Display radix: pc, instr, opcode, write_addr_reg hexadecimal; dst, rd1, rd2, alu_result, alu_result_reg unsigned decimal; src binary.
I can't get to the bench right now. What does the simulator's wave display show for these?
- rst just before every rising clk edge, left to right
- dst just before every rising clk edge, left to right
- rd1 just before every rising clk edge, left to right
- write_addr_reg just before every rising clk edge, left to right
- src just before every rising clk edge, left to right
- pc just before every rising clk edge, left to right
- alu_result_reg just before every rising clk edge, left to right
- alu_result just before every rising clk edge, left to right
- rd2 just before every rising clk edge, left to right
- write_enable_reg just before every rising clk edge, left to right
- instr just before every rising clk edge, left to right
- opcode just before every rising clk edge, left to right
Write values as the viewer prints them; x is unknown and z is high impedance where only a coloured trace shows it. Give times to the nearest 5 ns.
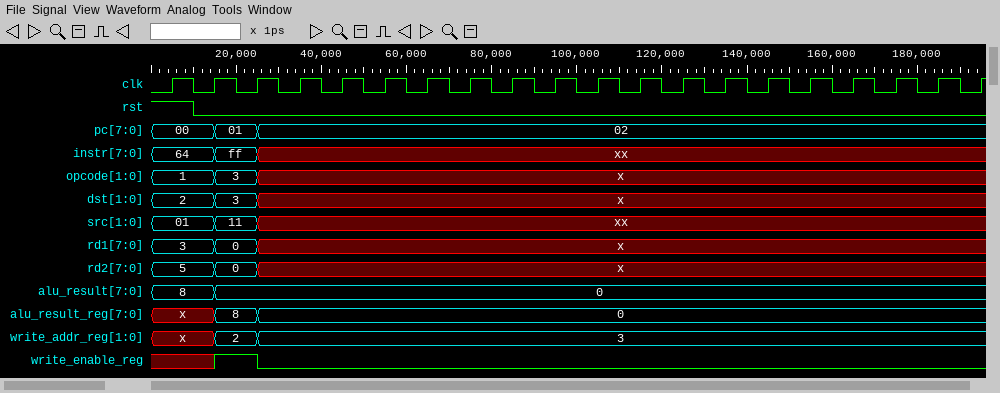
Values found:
1 0 0 0 0 0 0 0 0 0 0 0 0 0 0 0 0 0 0 0
2, 2, 3, x, x, x, x, x, x, x, x, x, x, x, x, x, x, x, x, x
3, 3, 0, x, x, x, x, x, x, x, x, x, x, x, x, x, x, x, x, x
x, x, 2, 3, 3, 3, 3, 3, 3, 3, 3, 3, 3, 3, 3, 3, 3, 3, 3, 3
01, 01, 11, xx, xx, xx, xx, xx, xx, xx, xx, xx, xx, xx, xx, xx, xx, xx, xx, xx
00, 00, 01, 02, 02, 02, 02, 02, 02, 02, 02, 02, 02, 02, 02, 02, 02, 02, 02, 02
x, x, 8, 0, 0, 0, 0, 0, 0, 0, 0, 0, 0, 0, 0, 0, 0, 0, 0, 0
8, 8, 0, 0, 0, 0, 0, 0, 0, 0, 0, 0, 0, 0, 0, 0, 0, 0, 0, 0
5, 5, 0, x, x, x, x, x, x, x, x, x, x, x, x, x, x, x, x, x
x x 1 0 0 0 0 0 0 0 0 0 0 0 0 0 0 0 0 0
64, 64, ff, xx, xx, xx, xx, xx, xx, xx, xx, xx, xx, xx, xx, xx, xx, xx, xx, xx
1, 1, 3, x, x, x, x, x, x, x, x, x, x, x, x, x, x, x, x, x
